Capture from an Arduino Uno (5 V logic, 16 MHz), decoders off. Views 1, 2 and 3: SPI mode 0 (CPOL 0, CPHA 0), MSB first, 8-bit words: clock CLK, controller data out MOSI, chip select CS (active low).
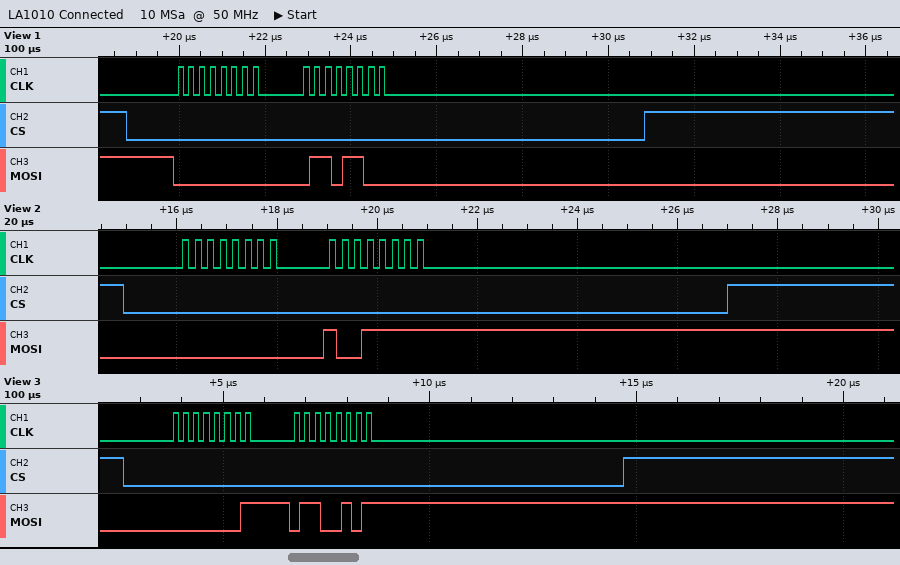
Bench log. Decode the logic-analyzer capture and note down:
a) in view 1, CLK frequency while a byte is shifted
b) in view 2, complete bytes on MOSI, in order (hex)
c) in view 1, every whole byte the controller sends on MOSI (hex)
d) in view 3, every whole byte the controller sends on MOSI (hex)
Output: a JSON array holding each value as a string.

["4 MHz", "0x00 0x9F", "00 6C", "01 65"]
